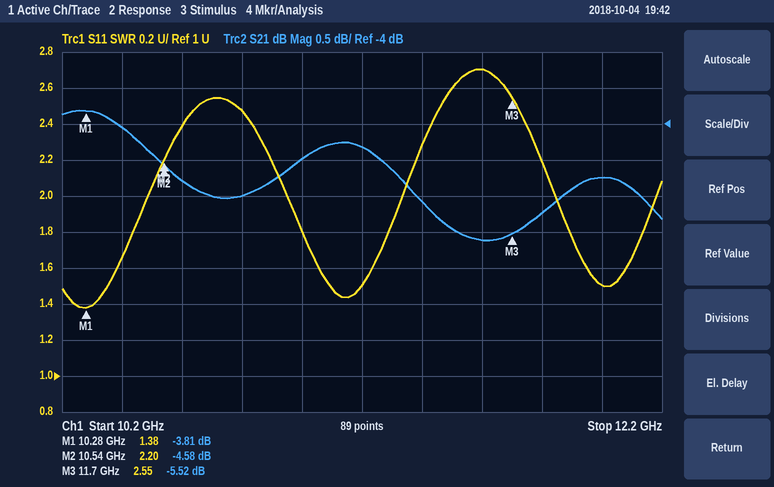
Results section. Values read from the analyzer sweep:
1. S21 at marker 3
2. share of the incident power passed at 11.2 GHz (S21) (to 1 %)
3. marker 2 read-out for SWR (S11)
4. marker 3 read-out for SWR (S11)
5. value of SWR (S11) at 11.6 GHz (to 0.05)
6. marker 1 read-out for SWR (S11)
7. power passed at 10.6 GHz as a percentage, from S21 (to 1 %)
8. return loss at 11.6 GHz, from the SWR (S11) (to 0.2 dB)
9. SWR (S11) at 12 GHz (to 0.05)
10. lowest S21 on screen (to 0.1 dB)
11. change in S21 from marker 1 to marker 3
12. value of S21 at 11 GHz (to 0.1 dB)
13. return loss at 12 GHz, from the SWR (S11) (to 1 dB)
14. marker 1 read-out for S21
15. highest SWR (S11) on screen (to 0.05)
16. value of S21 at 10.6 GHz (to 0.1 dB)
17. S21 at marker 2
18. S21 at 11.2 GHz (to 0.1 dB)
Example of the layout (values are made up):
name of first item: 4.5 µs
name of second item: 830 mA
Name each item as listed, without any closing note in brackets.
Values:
S21 at marker 3: -5.52 dB
share of the incident power passed at 11.2 GHz (S21): 37 %
marker 2 read-out for SWR: 2.20
marker 3 read-out for SWR: 2.55
value of SWR (S11) at 11.6 GHz: 2.70
marker 1 read-out for SWR: 1.38
power passed at 10.6 GHz as a percentage, from S21: 33 %
return loss at 11.6 GHz, from the SWR (S11): 6.8 dB
SWR (S11) at 12 GHz: 1.50
lowest S21 on screen: -5.6 dB
change in S21 from marker 1 to marker 3: -1.71 dB
value of S21 at 11 GHz: -4.5 dB
return loss at 12 GHz, from the SWR (S11): 14 dB
marker 1 read-out for S21: -3.81 dB
highest SWR (S11) on screen: 2.70
value of S21 at 10.6 GHz: -4.8 dB
S21 at marker 2: -4.58 dB
S21 at 11.2 GHz: -4.3 dB
